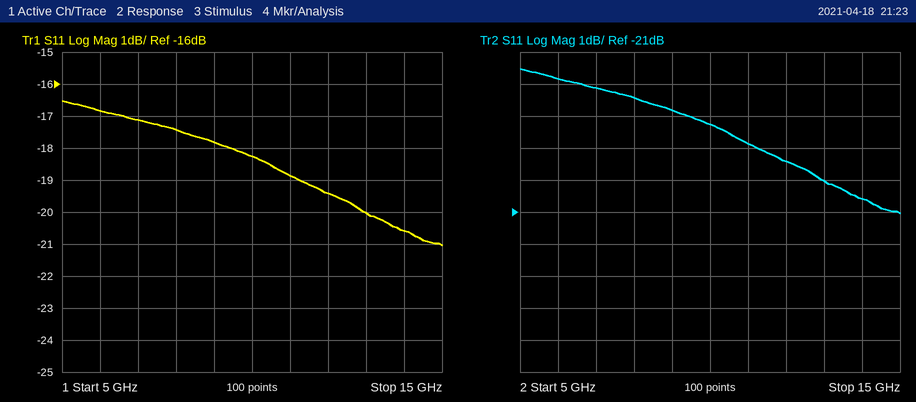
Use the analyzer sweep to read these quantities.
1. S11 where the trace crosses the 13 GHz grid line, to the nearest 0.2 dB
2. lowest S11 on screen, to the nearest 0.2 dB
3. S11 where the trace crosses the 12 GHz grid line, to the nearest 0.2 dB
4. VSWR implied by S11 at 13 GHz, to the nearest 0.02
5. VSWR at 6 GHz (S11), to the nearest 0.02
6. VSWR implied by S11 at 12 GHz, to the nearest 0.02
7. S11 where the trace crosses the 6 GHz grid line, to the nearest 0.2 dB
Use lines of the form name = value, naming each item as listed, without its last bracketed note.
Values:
S11 where the trace crosses the 13 GHz grid line, to the nearest 0.2 dB = -20.0 dB
lowest S11 on screen, to the nearest 0.2 dB = -21.0 dB
S11 where the trace crosses the 12 GHz grid line, to the nearest 0.2 dB = -19.4 dB
VSWR implied by S11 at 13 GHz, to the nearest 0.02 = 1.22
VSWR at 6 GHz (S11), to the nearest 0.02 = 1.34
VSWR implied by S11 at 12 GHz, to the nearest 0.02 = 1.24
S11 where the trace crosses the 6 GHz grid line, to the nearest 0.2 dB = -16.8 dB
